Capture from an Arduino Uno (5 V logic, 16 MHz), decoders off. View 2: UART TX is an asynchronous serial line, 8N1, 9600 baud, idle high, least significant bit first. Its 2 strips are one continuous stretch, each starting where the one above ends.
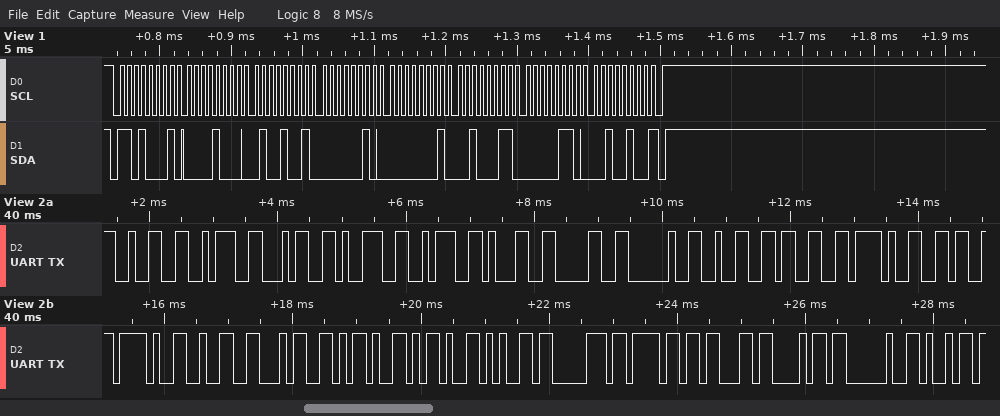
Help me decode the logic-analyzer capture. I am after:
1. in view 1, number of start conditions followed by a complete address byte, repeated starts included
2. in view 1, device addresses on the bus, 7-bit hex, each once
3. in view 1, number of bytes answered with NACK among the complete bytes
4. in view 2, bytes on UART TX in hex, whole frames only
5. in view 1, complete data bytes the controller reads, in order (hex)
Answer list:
1
0x68
1
32 3A 34 39 3A 31 30 20 32 33 2F 36 2F 32 34 2D 2D 65 70 6F 63 68 20 69
08 49 02 01 23 06 24
